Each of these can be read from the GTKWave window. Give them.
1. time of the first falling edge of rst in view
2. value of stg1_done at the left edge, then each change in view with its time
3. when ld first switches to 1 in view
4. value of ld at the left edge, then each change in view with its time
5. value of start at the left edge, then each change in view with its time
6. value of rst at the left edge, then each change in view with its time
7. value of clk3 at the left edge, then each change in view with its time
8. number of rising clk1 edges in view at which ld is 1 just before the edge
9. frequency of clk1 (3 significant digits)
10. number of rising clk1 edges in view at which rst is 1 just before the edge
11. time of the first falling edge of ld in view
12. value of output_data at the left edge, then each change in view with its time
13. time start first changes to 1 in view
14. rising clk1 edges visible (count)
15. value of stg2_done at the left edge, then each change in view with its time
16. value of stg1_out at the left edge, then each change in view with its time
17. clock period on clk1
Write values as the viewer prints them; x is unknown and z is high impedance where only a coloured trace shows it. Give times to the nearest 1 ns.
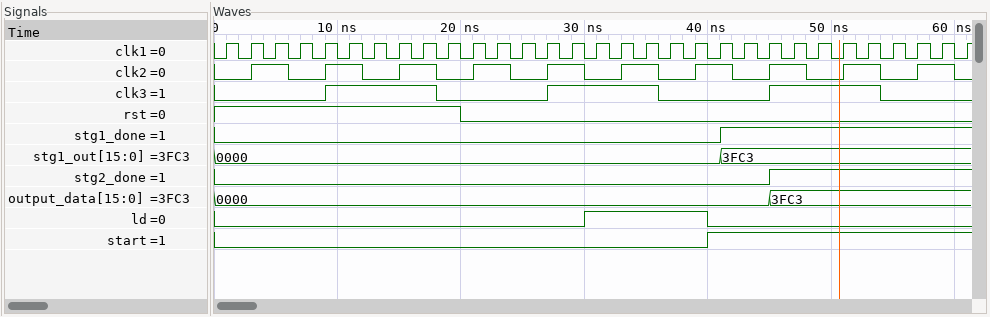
20 ns
0, 1 at 41 ns
30 ns
0, 1 at 30 ns, 0 at 40 ns
0, 1 at 40 ns
1, 0 at 20 ns
0, 1 at 9 ns, 0 at 18 ns, 1 at 27 ns, 0 at 36 ns, 1 at 45 ns, 0 at 54 ns
5
500 MHz
10
40 ns
0000, 3FC3 at 45 ns
40 ns
31
0, 1 at 45 ns
0000, 3FC3 at 41 ns
2 ns
